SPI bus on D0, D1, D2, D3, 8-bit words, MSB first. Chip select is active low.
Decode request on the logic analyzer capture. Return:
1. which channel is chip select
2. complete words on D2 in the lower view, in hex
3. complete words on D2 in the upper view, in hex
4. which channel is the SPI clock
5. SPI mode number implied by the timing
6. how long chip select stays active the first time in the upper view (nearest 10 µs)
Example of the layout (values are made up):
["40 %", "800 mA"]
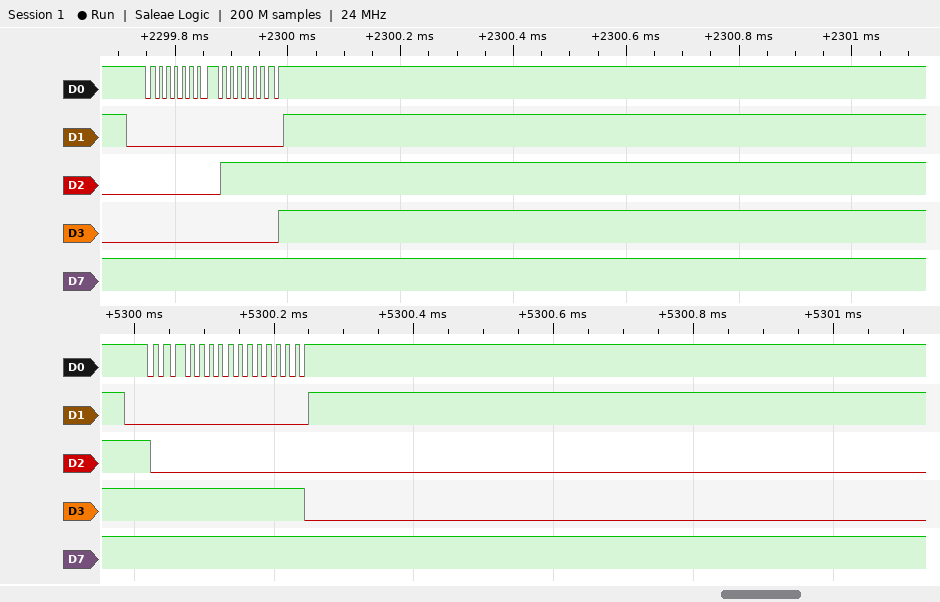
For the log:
["D1", "80, 00", "00, 7F", "D0", "2", "280 µs"]
